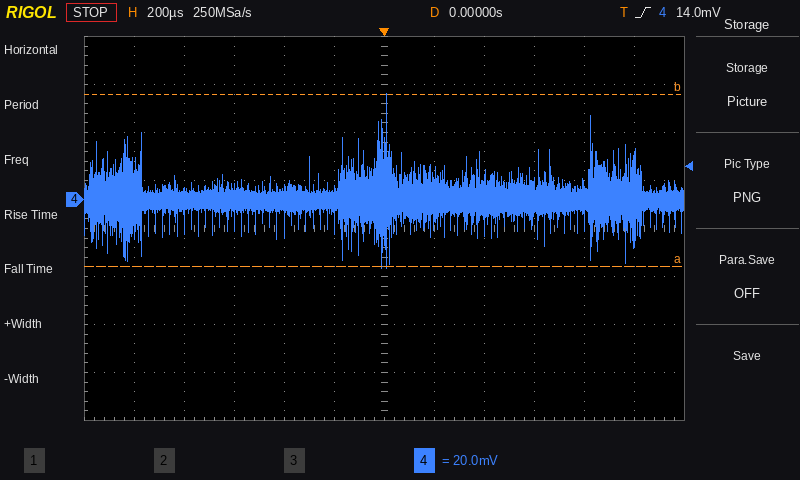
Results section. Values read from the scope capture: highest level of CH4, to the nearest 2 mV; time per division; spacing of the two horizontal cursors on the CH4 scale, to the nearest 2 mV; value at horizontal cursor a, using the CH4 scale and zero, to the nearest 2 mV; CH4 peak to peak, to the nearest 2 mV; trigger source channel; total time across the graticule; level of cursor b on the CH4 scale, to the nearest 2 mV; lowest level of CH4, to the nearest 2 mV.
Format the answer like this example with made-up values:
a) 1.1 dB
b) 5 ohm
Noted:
a) 44 mV
b) 200 µs
c) 72 mV
d) -28 mV
e) 72 mV
f) CH4
g) 2.4 ms
h) 44 mV
i) -28 mV
